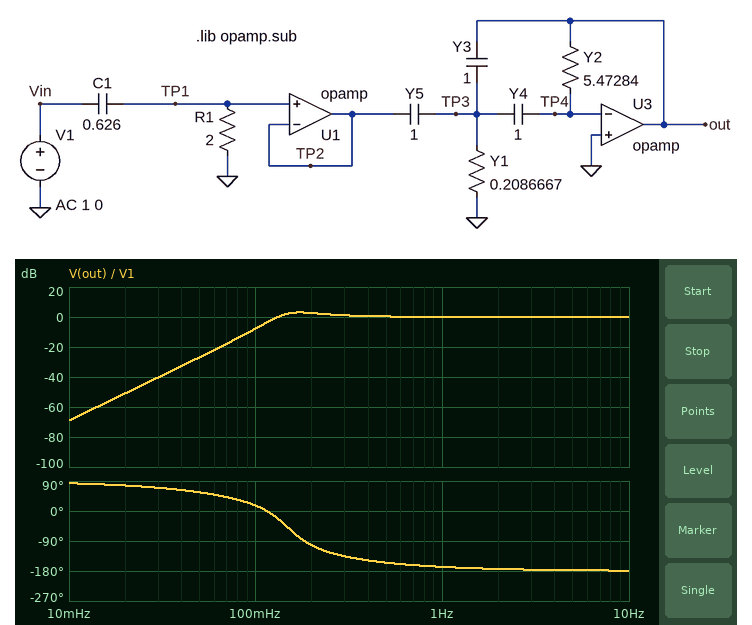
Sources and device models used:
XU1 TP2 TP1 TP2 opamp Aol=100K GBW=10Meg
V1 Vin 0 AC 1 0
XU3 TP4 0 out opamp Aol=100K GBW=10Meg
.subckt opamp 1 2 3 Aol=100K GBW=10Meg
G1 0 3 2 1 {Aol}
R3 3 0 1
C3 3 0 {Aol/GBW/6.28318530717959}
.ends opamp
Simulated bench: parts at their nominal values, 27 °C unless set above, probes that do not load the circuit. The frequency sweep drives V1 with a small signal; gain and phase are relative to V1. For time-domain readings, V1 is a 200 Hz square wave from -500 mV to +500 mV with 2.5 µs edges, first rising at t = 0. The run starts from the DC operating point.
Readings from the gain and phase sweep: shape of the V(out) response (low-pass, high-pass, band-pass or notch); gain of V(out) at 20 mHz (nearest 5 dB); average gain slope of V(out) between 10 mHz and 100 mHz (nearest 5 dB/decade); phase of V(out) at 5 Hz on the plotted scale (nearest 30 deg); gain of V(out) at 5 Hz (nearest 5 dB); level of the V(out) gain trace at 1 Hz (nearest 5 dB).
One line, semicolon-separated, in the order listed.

high-pass; -50 dB; 60 dB/decade; -180 deg; 0 dB; 0 dB
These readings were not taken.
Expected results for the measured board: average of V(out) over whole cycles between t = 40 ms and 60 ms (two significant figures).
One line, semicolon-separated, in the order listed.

-470 mV
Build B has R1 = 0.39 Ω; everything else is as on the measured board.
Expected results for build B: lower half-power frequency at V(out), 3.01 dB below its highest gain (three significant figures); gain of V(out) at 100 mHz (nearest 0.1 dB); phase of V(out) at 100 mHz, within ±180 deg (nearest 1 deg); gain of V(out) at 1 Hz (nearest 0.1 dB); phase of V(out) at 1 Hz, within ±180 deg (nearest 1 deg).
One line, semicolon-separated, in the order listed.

588 mHz; -19.9 dB; 46 deg; -1.4 dB; -142 deg
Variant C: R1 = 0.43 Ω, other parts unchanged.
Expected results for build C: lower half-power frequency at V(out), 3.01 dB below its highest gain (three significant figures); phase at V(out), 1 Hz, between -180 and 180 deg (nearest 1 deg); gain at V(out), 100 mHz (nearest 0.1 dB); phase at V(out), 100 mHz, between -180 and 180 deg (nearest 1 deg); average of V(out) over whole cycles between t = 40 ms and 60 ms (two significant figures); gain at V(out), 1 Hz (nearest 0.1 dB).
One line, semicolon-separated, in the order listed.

519 mHz; -144 deg; -19.1 dB; 45 deg; -400 mV; -1.1 dB
